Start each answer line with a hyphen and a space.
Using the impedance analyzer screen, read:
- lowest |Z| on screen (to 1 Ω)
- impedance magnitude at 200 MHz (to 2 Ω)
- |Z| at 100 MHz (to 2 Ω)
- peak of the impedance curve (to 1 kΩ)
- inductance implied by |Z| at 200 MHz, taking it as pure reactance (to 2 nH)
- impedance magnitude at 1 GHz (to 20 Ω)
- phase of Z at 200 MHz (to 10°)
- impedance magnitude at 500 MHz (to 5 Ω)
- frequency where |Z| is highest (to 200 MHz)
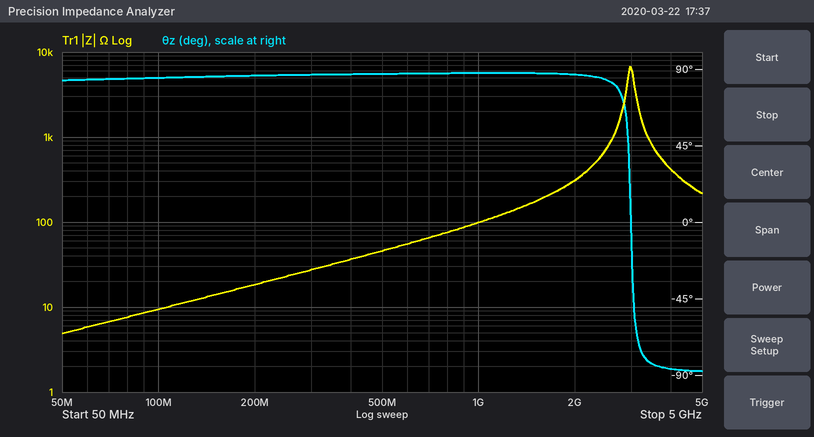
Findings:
- 5 Ω
- 18 Ω
- 10 Ω
- 7 kΩ
- 14 nH
- 100 Ω
- 90°
- 45 Ω
- 3.0 GHz
